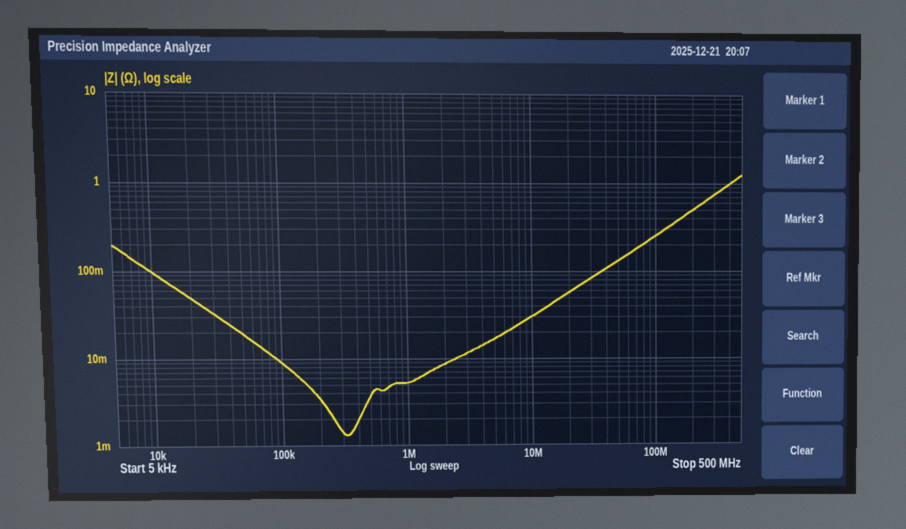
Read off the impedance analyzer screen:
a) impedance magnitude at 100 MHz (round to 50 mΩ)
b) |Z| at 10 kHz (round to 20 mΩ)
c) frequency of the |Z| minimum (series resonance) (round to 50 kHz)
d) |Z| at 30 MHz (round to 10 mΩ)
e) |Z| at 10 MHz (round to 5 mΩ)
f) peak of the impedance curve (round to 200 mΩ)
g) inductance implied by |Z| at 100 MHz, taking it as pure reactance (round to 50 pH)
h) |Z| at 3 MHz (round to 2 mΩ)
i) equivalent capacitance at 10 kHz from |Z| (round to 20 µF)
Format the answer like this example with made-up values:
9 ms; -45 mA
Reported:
250 mΩ; 100 mΩ; 300 kHz; 80 mΩ; 30 mΩ; 1.2 Ω; 400 pH; 12 mΩ; 160 µF
